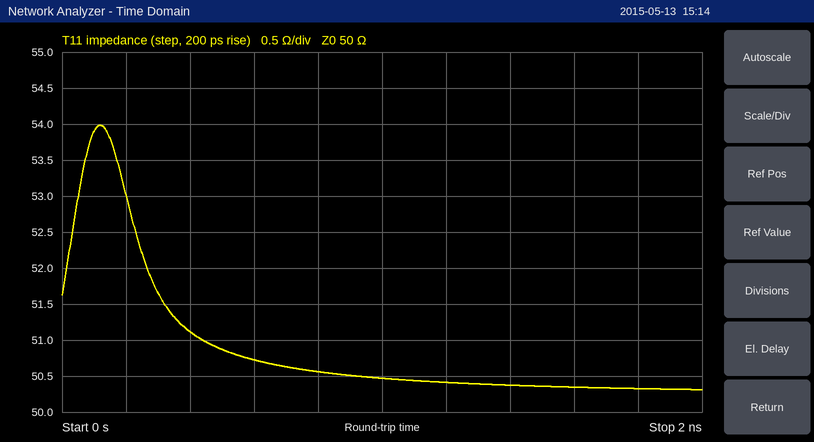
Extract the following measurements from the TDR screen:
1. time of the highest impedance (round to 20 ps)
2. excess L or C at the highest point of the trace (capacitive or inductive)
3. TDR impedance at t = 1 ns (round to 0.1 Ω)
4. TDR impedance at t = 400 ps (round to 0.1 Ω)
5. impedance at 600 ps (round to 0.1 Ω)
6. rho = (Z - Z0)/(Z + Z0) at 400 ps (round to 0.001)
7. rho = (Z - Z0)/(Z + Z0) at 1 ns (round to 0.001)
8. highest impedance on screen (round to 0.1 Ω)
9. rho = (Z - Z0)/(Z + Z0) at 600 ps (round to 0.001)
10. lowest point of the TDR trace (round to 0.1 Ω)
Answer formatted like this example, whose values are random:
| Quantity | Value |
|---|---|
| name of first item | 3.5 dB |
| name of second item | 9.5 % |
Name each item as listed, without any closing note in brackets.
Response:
| Quantity | Value |
|---|---|
| time of the highest impedance | 120 ps |
| excess L or C at the highest point of the trace | inductive |
| TDR impedance at t = 1 ns | 50.5 Ω |
| TDR impedance at t = 400 ps | 51.1 Ω |
| impedance at 600 ps | 50.7 Ω |
| rho = (Z - Z0)/(Z + Z0) at 400 ps | +0.011 |
| rho = (Z - Z0)/(Z + Z0) at 1 ns | +0.005 |
| highest impedance on screen | 54.0 Ω |
| rho = (Z - Z0)/(Z + Z0) at 600 ps | +0.007 |
| lowest point of the TDR trace | 50.3 Ω |
